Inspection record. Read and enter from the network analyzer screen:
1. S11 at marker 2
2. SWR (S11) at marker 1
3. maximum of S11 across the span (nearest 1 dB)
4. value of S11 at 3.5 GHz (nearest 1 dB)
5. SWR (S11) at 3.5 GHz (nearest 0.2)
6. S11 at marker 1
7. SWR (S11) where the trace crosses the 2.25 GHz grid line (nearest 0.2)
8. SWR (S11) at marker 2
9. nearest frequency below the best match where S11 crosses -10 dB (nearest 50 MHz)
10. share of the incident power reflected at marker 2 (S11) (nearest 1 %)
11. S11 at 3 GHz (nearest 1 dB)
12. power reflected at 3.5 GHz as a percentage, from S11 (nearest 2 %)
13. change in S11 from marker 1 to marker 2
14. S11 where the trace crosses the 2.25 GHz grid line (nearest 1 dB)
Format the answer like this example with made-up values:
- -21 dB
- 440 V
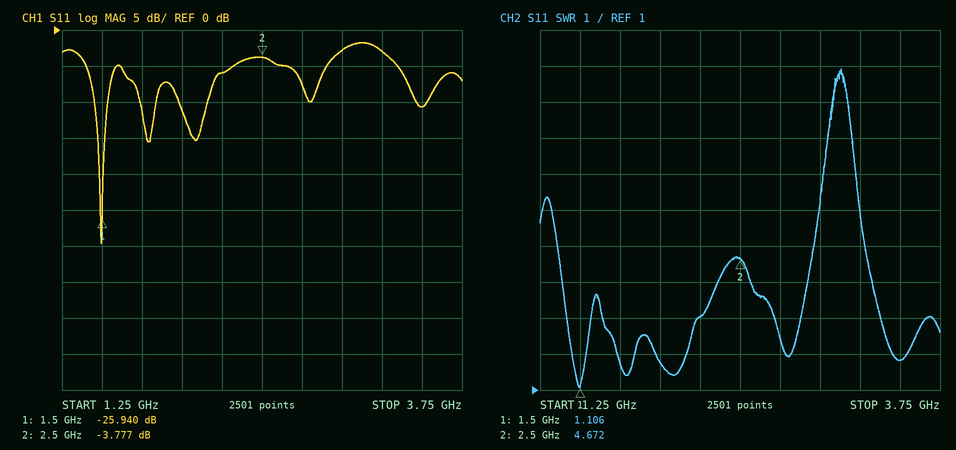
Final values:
- -3.777 dB
- 1.106
- -2 dB
- -11 dB
- 1.8
- -25.940 dB
- 3.0
- 4.672
- 1.45 GHz
- 42 %
- -3 dB
- 8 %
- 22.163 dB
- -6 dB
